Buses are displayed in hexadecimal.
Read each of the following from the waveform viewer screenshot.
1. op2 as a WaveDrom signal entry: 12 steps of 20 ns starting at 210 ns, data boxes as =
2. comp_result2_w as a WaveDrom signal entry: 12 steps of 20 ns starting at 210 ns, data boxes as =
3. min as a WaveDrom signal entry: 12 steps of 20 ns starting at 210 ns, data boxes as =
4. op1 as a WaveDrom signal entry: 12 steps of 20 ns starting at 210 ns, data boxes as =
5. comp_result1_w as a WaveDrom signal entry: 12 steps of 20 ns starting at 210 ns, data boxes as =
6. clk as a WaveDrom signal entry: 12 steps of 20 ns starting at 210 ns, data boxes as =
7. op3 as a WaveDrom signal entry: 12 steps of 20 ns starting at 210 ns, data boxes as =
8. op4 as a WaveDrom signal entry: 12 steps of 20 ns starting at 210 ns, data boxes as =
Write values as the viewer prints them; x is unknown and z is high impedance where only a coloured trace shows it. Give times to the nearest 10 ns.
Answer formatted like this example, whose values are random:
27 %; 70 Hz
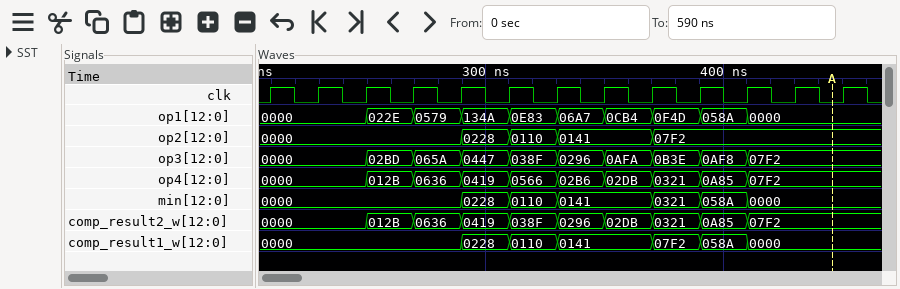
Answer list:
{name: 'op2', wave: '=...===.=...', data: '0000 0228 0110 0141 07F2'}; {name: 'comp_result2_w', wave: '=.=========.', data: '0000 012B 0636 0419 038F 0296 02DB 0321 0A85 07F2'}; {name: 'min', wave: '=...===.===.', data: '0000 0228 0110 0141 0321 058A 0000'}; {name: 'op1', wave: '=.=========.', data: '0000 022E 0579 134A 0E83 06A7 0CB4 0F4D 058A 0000'}; {name: 'comp_result1_w', wave: '=...===.===.', data: '0000 0228 0110 0141 07F2 058A 0000'}; {name: 'clk', wave: 'p...........'}; {name: 'op3', wave: '=.=========.', data: '0000 02BD 065A 0447 038F 0296 0AFA 0B3E 0AF8 07F2'}; {name: 'op4', wave: '=.=========.', data: '0000 012B 0636 0419 0566 02B6 02DB 0321 0A85 07F2'}
